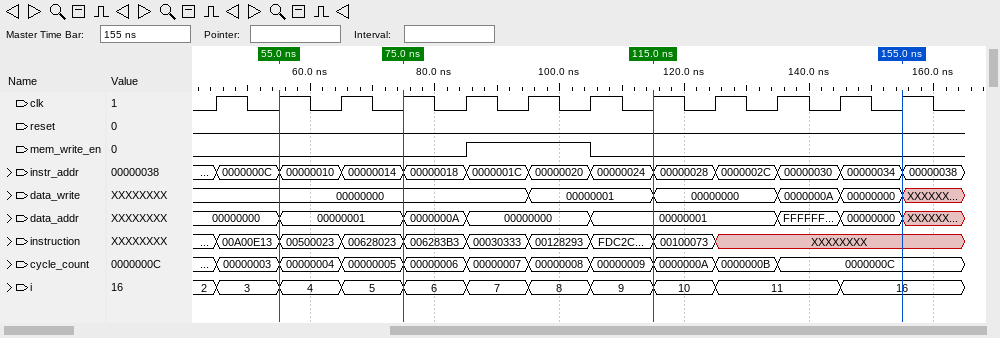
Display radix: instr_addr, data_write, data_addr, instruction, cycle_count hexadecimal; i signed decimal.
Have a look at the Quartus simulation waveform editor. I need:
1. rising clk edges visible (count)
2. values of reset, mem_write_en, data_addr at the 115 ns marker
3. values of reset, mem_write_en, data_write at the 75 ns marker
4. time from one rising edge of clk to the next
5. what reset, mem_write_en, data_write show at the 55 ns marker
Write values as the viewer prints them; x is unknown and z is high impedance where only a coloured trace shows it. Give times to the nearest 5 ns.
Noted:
12
reset=0, mem_write_en=0, data_addr=00000001
reset=0, mem_write_en=0, data_write=00000000
10 ns
reset=0, mem_write_en=0, data_write=00000000
